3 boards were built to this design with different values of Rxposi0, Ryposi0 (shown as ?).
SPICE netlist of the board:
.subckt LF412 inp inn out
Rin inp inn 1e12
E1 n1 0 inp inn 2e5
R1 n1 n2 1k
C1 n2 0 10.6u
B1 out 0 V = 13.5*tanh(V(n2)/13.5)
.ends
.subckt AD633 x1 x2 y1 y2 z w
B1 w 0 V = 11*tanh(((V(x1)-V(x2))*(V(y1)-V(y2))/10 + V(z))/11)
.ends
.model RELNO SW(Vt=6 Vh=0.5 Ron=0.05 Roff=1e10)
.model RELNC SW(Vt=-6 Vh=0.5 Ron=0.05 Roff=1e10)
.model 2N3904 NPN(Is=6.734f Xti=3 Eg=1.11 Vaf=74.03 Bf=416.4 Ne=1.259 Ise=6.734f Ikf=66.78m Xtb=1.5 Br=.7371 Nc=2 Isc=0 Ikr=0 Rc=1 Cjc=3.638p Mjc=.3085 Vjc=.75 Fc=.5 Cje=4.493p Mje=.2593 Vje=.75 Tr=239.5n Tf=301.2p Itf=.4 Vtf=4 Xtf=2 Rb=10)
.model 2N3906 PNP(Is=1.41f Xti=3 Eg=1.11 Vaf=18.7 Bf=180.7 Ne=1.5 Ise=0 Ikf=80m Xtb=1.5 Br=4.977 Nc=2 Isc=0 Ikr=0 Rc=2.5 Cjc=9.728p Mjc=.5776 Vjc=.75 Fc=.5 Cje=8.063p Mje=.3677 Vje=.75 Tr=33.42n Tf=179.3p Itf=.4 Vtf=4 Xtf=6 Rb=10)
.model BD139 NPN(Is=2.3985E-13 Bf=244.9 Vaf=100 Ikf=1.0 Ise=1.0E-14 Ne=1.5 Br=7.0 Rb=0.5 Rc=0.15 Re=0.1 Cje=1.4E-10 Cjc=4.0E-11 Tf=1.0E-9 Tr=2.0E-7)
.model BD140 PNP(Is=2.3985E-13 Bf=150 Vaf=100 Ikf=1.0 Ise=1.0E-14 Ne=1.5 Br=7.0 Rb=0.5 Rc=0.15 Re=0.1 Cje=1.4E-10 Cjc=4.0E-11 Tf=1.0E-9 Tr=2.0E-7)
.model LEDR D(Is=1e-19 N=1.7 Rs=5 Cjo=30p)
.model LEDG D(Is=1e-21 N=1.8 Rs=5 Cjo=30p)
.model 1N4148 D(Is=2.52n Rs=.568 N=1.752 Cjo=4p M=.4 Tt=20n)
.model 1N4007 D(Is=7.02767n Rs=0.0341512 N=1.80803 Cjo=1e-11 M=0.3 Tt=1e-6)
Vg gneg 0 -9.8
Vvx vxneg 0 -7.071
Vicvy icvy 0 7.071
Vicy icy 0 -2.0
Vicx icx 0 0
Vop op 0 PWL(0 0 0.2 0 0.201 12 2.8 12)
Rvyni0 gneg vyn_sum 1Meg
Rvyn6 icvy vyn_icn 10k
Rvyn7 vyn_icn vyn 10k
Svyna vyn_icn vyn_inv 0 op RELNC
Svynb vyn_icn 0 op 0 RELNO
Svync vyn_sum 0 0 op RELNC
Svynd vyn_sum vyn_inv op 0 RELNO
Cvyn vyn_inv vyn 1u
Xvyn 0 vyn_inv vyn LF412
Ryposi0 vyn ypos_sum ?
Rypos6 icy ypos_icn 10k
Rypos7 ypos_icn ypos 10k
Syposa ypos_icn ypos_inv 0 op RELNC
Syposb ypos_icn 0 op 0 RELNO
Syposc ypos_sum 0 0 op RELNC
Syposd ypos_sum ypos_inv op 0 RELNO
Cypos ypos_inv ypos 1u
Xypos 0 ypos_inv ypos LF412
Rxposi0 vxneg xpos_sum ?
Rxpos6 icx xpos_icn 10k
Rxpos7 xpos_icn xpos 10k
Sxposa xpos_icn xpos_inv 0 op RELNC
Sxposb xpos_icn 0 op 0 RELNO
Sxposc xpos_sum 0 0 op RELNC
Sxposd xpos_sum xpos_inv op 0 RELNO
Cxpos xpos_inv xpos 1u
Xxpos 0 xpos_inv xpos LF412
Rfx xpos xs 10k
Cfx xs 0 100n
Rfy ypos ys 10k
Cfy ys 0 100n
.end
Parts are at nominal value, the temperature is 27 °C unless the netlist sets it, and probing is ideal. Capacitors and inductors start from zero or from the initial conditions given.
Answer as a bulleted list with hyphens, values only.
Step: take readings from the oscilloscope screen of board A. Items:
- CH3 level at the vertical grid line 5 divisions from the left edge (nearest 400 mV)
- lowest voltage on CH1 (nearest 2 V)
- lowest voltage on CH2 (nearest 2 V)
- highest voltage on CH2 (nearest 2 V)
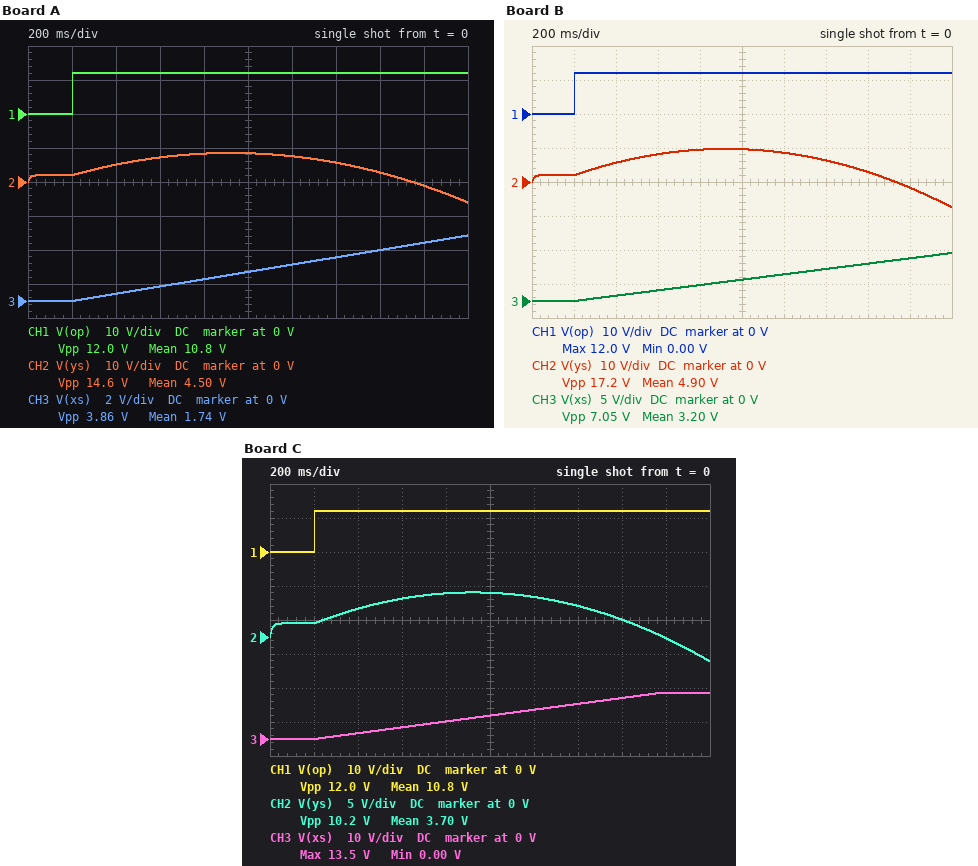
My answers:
- 1.6 V
- 0 V
- -6 V
- 8 V
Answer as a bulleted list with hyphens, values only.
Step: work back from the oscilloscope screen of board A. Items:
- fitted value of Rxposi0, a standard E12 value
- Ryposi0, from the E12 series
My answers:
- 3.3 MΩ
- 390 kΩ
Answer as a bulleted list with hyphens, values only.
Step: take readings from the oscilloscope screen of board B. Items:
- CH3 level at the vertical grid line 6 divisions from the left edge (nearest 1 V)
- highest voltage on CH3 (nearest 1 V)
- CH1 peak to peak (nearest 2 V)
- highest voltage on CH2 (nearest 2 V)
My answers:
- 4 V
- 7 V
- 12 V
- 10 V
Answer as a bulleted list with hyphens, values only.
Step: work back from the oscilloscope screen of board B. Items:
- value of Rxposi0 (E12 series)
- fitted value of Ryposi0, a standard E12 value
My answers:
- 1.8 MΩ
- 330 kΩ
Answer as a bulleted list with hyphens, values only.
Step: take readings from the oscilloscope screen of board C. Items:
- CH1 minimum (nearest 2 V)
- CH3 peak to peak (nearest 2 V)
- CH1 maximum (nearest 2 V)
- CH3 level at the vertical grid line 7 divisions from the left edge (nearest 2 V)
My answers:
- 0 V
- 14 V
- 12 V
- 10 V
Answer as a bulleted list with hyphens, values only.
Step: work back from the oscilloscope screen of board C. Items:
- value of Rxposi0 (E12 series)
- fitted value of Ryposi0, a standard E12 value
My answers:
- 820 kΩ
- 560 kΩ
